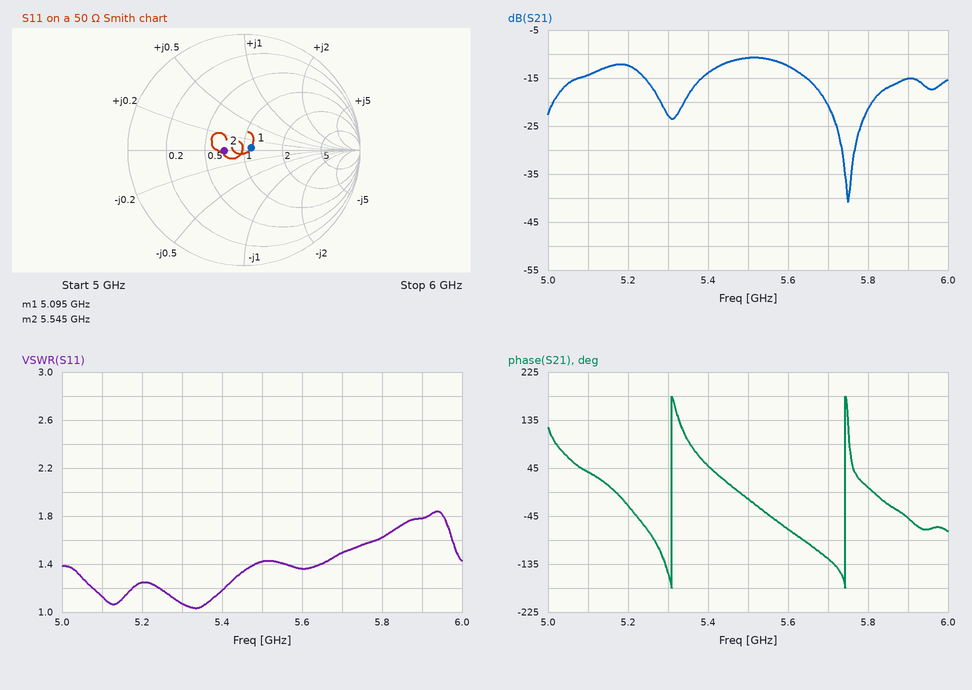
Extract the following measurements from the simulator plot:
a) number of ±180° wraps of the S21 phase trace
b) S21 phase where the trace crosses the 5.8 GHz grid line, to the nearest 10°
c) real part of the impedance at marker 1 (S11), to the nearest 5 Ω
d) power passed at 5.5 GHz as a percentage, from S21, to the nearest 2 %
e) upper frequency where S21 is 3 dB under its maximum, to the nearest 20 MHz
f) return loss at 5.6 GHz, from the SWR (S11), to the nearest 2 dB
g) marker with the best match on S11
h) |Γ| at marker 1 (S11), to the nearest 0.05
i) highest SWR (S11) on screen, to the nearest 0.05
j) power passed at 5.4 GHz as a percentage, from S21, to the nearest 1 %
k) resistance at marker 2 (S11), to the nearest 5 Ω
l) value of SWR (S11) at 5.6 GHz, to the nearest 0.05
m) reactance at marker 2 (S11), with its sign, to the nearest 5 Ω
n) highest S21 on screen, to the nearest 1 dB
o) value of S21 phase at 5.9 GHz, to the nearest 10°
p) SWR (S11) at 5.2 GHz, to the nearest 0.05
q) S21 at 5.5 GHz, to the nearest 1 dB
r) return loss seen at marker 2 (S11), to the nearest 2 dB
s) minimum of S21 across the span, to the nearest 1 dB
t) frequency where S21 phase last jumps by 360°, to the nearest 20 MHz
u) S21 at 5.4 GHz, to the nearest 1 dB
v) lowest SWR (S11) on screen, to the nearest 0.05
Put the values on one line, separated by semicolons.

2; 10°; 55 Ω; 8 %; 5.62 GHz; 16 dB; marker 1; 0.05; 1.85; 4 %; 35 Ω; 1.35; 0 Ω; -11 dB; -50°; 1.25; -11 dB; 16 dB; -41 dB; 5.74 GHz; -14 dB; 1.05
